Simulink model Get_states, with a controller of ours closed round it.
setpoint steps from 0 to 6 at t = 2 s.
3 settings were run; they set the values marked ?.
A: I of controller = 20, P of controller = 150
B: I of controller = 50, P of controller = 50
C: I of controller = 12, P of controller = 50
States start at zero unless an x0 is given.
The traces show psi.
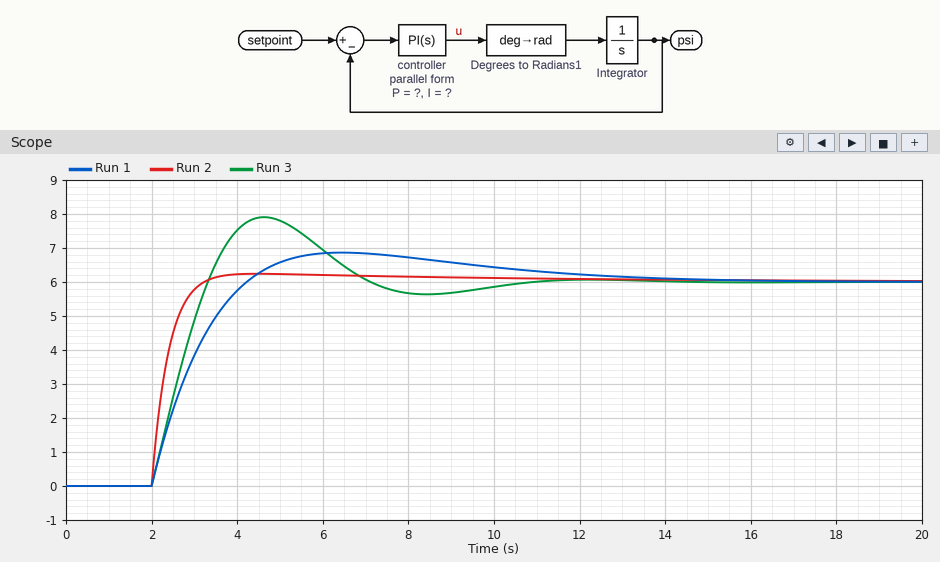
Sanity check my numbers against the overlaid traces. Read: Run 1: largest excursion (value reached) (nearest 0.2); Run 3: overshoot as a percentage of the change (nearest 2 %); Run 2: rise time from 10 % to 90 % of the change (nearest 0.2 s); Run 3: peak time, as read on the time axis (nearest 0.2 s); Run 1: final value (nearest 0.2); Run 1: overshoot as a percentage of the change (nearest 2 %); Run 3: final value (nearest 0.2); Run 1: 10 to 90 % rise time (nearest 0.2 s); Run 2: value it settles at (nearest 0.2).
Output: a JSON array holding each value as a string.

["6.8", "32 %", "0.8 s", "4.6 s", "6.0", "14 %", "6.0", "1.6 s", "6.0"]
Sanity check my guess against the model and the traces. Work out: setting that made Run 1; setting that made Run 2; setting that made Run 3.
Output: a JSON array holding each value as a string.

["C", "A", "B"]
